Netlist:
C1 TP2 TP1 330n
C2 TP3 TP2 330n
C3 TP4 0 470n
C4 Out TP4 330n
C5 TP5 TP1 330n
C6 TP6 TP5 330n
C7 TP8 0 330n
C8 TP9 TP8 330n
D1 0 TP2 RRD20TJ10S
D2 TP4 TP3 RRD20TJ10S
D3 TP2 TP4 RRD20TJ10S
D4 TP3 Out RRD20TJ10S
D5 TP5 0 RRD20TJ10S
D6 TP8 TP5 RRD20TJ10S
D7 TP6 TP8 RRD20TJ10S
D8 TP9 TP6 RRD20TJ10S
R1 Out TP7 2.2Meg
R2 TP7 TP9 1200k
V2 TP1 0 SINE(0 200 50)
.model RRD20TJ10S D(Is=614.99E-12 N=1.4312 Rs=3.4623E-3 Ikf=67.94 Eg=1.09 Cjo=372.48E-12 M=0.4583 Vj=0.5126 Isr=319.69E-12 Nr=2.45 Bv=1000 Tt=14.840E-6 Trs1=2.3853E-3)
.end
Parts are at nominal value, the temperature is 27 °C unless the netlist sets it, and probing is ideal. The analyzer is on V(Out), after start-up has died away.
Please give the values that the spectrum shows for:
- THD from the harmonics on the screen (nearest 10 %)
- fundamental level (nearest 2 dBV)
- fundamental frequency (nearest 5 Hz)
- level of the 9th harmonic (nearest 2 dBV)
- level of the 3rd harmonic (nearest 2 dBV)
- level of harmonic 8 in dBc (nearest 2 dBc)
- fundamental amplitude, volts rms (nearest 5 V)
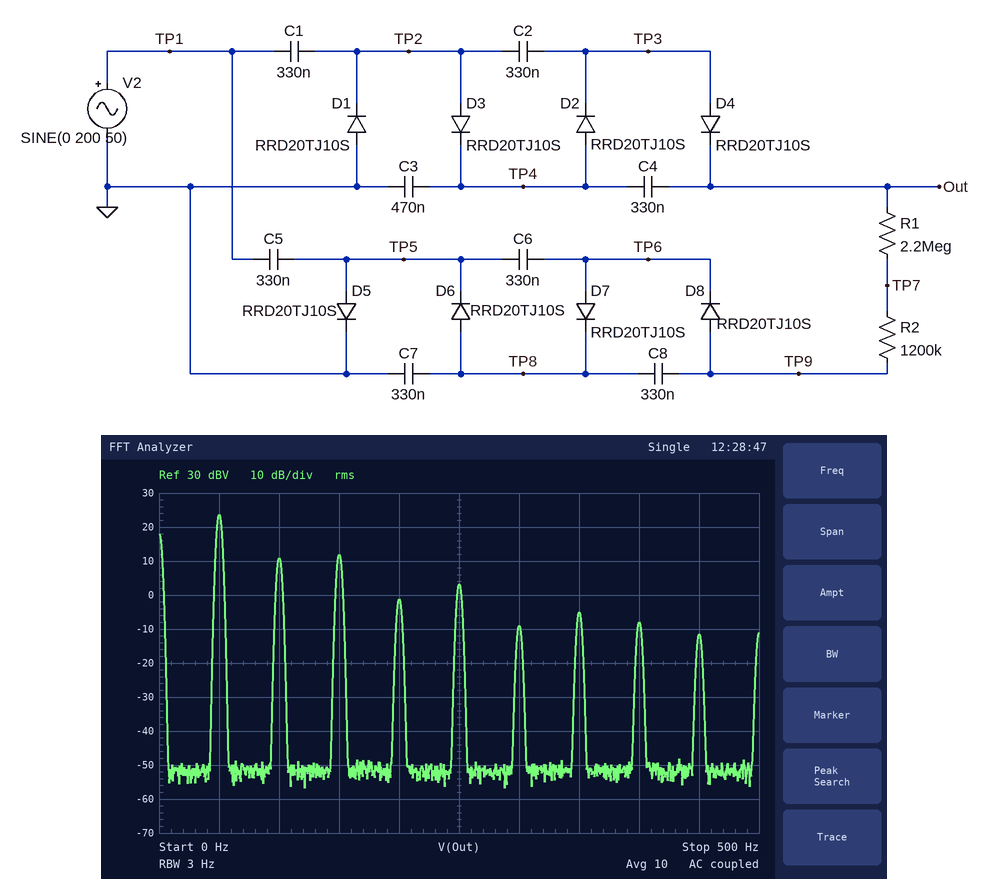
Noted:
40 %
24 dBV
50 Hz
-12 dBV
12 dBV
-32 dBc
15 V
